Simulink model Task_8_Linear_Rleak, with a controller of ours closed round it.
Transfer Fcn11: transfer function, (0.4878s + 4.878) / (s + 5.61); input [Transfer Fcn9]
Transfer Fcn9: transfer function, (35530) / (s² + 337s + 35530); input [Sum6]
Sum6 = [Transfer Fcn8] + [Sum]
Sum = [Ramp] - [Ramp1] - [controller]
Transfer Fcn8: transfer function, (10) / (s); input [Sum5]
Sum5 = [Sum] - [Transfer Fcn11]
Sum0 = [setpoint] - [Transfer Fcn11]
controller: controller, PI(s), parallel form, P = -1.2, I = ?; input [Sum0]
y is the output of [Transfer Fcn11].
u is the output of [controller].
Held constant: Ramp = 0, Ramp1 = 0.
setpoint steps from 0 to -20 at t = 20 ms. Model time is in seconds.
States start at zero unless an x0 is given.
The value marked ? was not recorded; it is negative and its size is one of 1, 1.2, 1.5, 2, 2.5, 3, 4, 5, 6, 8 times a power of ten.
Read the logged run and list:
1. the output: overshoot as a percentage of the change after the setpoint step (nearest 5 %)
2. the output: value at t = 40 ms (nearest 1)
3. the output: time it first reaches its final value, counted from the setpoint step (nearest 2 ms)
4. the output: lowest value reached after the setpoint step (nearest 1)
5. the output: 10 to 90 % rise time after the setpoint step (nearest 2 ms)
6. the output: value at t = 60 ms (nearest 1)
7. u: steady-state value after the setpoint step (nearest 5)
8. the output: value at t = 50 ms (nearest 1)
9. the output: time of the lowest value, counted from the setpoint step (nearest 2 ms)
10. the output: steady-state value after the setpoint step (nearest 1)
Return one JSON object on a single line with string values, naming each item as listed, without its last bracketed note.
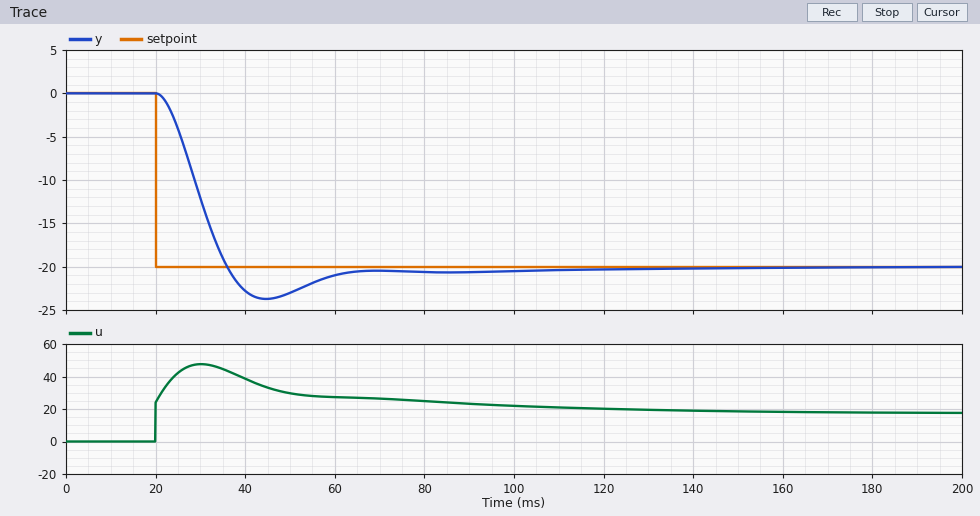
{"the output: overshoot as a percentage of the change after the setpoint step": "20 %", "the output: value at t = 40 ms": "-23", "the output: time it first reaches its final value, counted from the setpoint step": "16 ms", "the output: lowest value reached after the setpoint step": "-24", "the output: 10 to 90 % rise time after the setpoint step": "10 ms", "the output: value at t = 60 ms": "-21", "u: steady-state value after the setpoint step": "20", "the output: value at t = 50 ms": "-23", "the output: time of the lowest value, counted from the setpoint step": "24 ms", "the output: steady-state value after the setpoint step": "-20"}
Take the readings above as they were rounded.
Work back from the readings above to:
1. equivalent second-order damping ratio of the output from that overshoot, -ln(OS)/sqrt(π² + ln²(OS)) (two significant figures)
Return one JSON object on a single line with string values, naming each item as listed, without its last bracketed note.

{"equivalent second-order damping ratio of the output from that overshoot, -ln(OS)/sqrt(π² + ln²(OS))": "0.46"}
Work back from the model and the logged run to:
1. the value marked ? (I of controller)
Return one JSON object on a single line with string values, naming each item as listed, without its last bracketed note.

{"the value marked ?": "-250"}
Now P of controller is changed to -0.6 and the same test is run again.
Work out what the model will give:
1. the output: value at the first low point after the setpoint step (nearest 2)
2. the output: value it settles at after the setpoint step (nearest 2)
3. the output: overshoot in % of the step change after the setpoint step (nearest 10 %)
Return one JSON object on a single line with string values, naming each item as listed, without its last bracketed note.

{"the output: value at the first low point after the setpoint step": "-26", "the output: value it settles at after the setpoint step": "-20", "the output: overshoot in % of the step change after the setpoint step": "30 %"}
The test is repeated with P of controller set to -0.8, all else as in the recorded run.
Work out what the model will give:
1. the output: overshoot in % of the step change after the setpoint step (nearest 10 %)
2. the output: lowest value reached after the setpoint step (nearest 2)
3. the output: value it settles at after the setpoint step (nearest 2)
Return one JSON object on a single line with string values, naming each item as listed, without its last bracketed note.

{"the output: overshoot in % of the step change after the setpoint step": "30 %", "the output: lowest value reached after the setpoint step": "-26", "the output: value it settles at after the setpoint step": "-20"}
